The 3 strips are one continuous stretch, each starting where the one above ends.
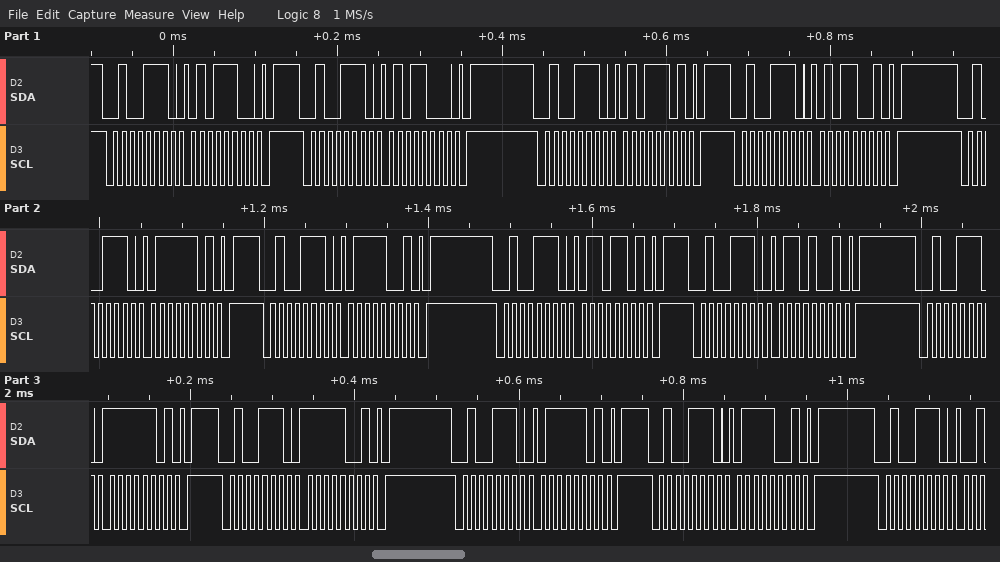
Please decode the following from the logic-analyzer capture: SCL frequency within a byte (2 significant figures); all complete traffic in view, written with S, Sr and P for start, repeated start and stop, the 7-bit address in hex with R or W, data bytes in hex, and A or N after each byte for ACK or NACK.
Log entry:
100 kHz
S 27W A 5C A P S 27W A 58 A P S 27W A 5D A P S 27W A 59 A P S 27W A 7D A P S 27W A 79 A P S 27W A 6D A P S 27W A 69 A P S 27W A FD A P S 27W A F9 A P S 27W A 7D A P S 27W A 79 A P S 27W A
